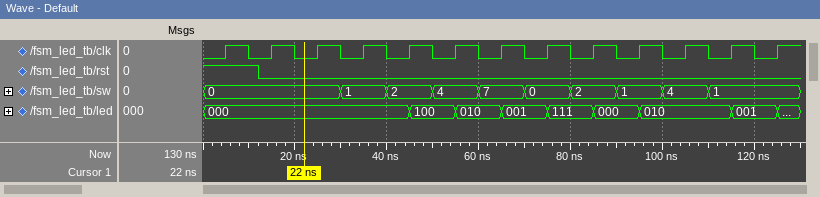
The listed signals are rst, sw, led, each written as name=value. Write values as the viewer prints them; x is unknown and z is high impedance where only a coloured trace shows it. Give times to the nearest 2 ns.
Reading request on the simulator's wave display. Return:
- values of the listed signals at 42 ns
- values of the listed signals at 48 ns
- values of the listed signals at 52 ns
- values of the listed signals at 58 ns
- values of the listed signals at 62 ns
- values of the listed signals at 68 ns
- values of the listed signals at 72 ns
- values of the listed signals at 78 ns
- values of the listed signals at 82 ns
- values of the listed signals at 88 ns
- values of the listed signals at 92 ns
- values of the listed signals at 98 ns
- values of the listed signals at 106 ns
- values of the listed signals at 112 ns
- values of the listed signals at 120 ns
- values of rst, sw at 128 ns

rst=0, sw=2, led=000
rst=0, sw=2, led=100
rst=0, sw=4, led=100
rst=0, sw=4, led=010
rst=0, sw=7, led=010
rst=0, sw=7, led=001
rst=0, sw=0, led=001
rst=0, sw=0, led=111
rst=0, sw=2, led=111
rst=0, sw=2, led=000
rst=0, sw=1, led=000
rst=0, sw=1, led=010
rst=0, sw=4, led=010
rst=0, sw=1, led=010
rst=0, sw=1, led=001
rst=0, sw=1
